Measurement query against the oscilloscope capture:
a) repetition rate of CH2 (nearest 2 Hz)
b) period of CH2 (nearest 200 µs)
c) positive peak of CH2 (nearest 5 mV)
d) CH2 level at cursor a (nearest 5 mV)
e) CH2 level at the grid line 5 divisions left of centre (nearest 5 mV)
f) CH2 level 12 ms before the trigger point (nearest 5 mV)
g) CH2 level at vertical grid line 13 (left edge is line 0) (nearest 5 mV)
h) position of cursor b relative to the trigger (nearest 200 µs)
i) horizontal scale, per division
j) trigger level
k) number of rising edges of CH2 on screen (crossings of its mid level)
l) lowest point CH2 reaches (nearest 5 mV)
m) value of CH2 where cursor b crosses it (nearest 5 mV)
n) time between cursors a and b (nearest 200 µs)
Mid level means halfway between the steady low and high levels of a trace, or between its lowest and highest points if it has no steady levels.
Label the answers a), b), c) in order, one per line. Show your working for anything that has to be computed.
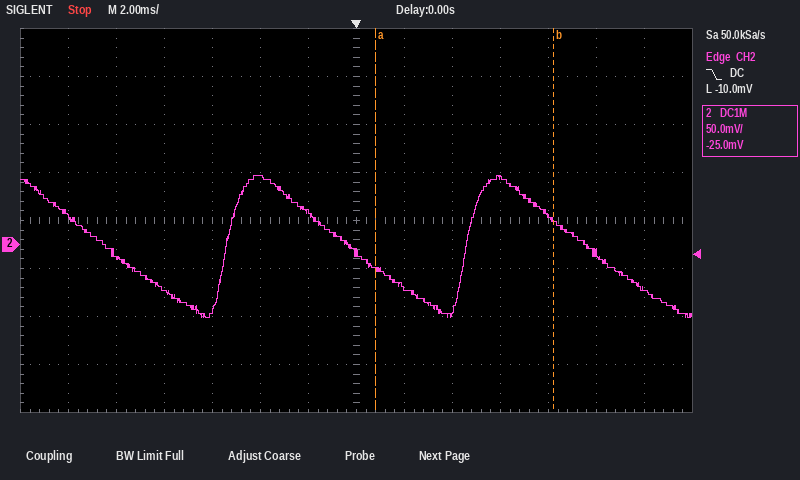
a) 1 / 10.0 ms ≈ 100 Hz
b) 10.0 ms
c) 70 mV
d) -25 mV
e) -15 mV
f) 30 mV
g) -45 mV
h) +8.2 ms
i) 2 ms
j) -10.0 mV
k) 2
l) -75 mV
m) 25 mV
n) 7.4 ms
